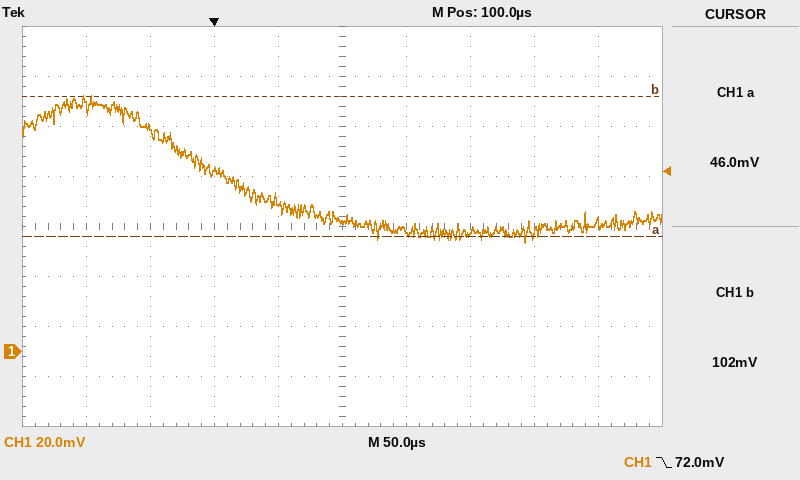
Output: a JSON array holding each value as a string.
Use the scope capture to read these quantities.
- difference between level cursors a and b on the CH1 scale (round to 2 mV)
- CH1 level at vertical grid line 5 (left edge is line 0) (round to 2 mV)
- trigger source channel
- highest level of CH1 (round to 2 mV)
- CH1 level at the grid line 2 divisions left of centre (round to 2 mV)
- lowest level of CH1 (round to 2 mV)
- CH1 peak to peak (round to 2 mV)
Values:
["56 mV", "52 mV", "CH1", "102 mV", "72 mV", "44 mV", "58 mV"]
